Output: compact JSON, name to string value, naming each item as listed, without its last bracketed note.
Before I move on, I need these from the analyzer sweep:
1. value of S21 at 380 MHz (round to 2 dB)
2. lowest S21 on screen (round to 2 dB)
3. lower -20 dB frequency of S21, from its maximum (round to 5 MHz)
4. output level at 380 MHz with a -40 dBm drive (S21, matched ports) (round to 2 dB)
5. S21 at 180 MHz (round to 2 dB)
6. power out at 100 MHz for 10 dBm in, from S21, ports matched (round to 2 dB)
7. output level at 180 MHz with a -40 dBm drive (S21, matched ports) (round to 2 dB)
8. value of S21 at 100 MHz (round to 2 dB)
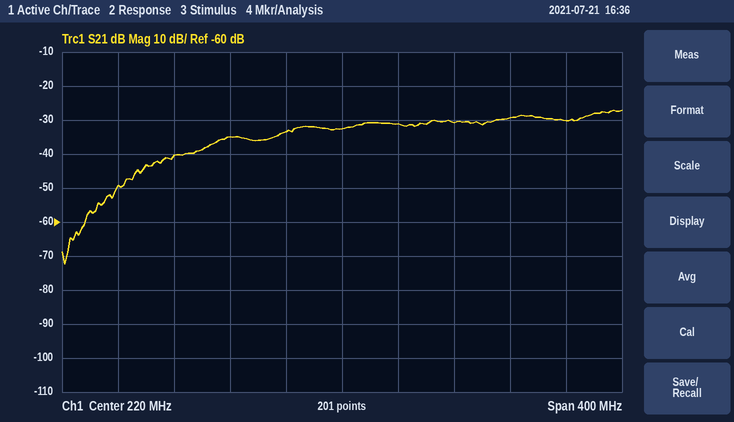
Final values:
{"value of S21 at 380 MHz": "-30 dB", "lowest S21 on screen": "-72 dB", "lower -20 dB frequency of S21, from its maximum": "70 MHz", "output level at 380 MHz with a -40 dBm drive (S21, matched ports)": "-70 dBm", "S21 at 180 MHz": "-34 dB", "power out at 100 MHz for 10 dBm in, from S21, ports matched": "-30 dBm", "output level at 180 MHz with a -40 dBm drive (S21, matched ports)": "-74 dBm", "value of S21 at 100 MHz": "-40 dB"}
